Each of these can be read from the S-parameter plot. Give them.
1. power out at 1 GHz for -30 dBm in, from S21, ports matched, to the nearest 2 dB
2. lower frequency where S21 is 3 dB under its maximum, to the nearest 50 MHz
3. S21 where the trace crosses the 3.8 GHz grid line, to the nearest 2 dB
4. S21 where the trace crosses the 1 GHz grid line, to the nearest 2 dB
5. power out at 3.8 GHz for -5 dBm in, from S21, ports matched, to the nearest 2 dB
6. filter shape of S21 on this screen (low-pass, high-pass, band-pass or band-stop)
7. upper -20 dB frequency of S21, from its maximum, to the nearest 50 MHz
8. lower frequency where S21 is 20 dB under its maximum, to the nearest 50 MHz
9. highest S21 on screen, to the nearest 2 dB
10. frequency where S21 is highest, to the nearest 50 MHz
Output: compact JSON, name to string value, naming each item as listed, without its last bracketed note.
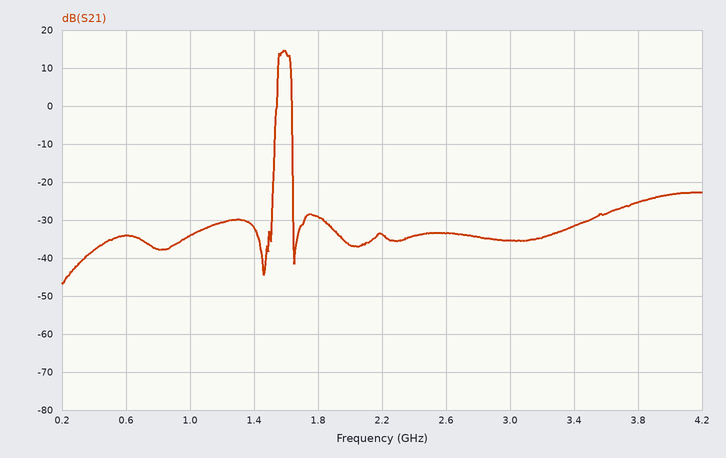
{"power out at 1 GHz for -30 dBm in, from S21, ports matched, to the nearest 2 dB": "-64 dBm", "lower frequency where S21 is 3 dB under its maximum, to the nearest 50 MHz": "1.55 GHz", "S21 where the trace crosses the 3.8 GHz grid line, to the nearest 2 dB": "-26 dB", "S21 where the trace crosses the 1 GHz grid line, to the nearest 2 dB": "-34 dB", "power out at 3.8 GHz for -5 dBm in, from S21, ports matched, to the nearest 2 dB": "-30 dBm", "filter shape of S21 on this screen": "band-pass", "upper -20 dB frequency of S21, from its maximum, to the nearest 50 MHz": "1.65 GHz", "lower frequency where S21 is 20 dB under its maximum, to the nearest 50 MHz": "1.55 GHz", "highest S21 on screen, to the nearest 2 dB": "14 dB", "frequency where S21 is highest, to the nearest 50 MHz": "1.60 GHz"}
